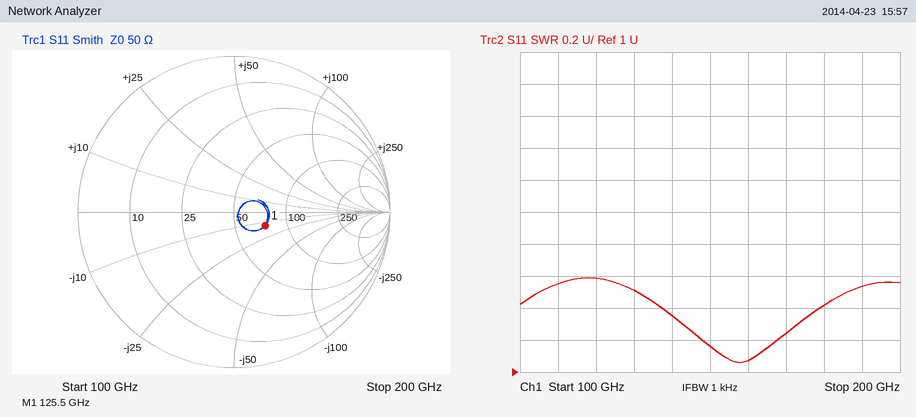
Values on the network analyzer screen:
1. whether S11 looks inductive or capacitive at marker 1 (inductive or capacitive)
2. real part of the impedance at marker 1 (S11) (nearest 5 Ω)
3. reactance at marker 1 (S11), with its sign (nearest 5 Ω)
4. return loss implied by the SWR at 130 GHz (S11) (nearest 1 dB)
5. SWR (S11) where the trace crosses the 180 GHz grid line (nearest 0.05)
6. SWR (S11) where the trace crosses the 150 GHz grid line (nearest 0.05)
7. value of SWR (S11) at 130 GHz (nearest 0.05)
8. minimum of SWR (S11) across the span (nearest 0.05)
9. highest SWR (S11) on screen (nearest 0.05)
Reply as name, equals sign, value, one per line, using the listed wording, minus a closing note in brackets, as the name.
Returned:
whether S11 looks inductive or capacitive at marker 1 = capacitive
real part of the impedance at marker 1 (S11) = 75 Ω
reactance at marker 1 (S11), with its sign = -15 Ω
return loss implied by the SWR at 130 GHz (S11) = 14 dB
SWR (S11) where the trace crosses the 180 GHz grid line = 1.40
SWR (S11) where the trace crosses the 150 GHz grid line = 1.15
value of SWR (S11) at 130 GHz = 1.50
minimum of SWR (S11) across the span = 1.05
highest SWR (S11) on screen = 1.60
